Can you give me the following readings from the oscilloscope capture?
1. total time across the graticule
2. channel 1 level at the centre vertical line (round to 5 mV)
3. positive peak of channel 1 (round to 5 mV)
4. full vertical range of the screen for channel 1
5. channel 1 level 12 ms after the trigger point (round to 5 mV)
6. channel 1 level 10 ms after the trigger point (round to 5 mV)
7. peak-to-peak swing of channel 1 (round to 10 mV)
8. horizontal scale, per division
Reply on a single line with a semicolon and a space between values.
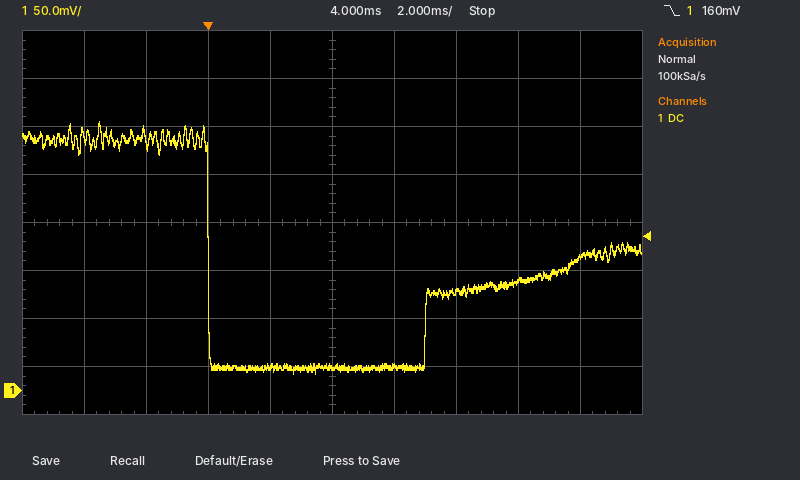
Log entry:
20 ms; 25 mV; 280 mV; 400 mV; 140 mV; 115 mV; 260 mV; 2 ms
